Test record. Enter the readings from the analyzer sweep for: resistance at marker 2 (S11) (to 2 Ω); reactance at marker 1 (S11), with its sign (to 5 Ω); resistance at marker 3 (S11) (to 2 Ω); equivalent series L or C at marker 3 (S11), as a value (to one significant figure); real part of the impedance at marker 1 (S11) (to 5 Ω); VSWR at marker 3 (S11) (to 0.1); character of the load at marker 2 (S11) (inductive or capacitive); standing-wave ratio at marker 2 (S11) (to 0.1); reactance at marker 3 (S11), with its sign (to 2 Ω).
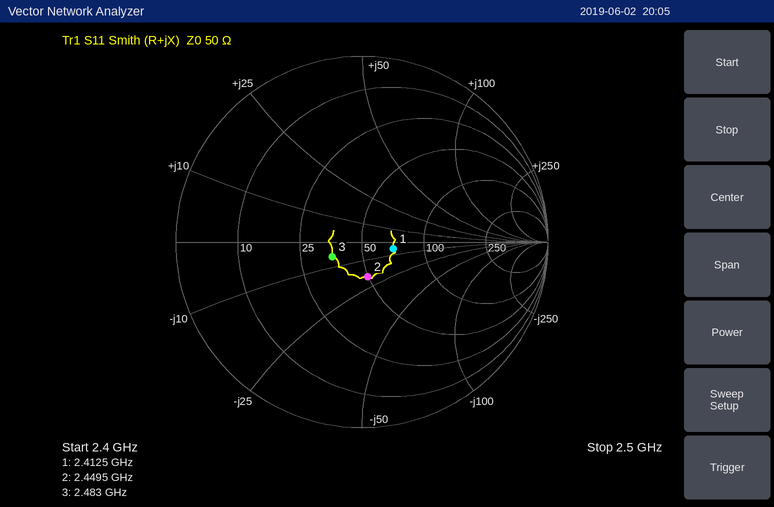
50 Ω
-5 Ω
36 Ω
10 pF
70 Ω
1.4
capacitive
1.5
-6 Ω
